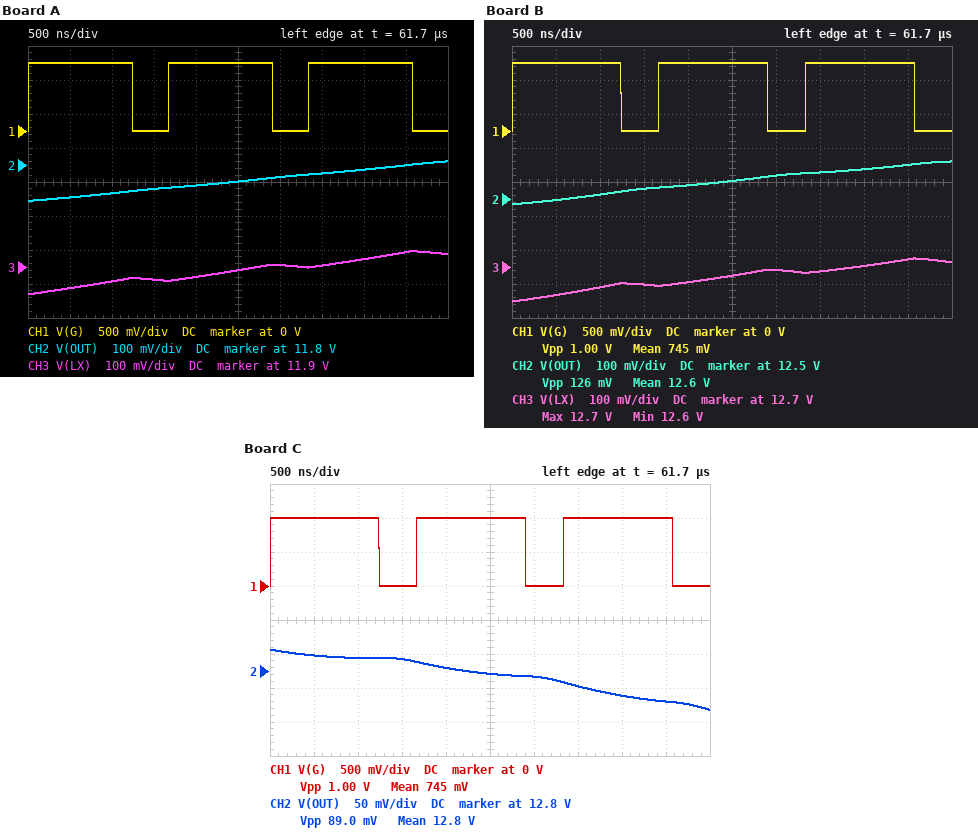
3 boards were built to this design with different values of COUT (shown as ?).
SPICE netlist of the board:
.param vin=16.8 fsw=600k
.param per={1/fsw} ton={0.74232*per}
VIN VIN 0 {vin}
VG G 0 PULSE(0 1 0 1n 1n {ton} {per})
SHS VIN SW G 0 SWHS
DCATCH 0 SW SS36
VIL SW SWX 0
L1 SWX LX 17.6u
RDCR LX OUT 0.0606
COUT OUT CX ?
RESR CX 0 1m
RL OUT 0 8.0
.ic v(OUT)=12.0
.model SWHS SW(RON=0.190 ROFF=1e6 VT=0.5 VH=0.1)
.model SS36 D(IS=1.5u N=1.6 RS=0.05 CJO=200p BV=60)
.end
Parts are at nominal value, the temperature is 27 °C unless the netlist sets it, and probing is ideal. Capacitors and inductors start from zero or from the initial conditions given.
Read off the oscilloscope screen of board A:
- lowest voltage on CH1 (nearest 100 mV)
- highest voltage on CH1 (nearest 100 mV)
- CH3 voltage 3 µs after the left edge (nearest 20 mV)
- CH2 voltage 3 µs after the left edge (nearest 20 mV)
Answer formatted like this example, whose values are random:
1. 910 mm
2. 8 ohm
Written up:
1. 0 V
2. 1.0 V
3. 11.90 V
4. 11.76 V
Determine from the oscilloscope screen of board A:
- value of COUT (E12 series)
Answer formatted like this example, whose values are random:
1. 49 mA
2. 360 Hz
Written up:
1. 33 µF
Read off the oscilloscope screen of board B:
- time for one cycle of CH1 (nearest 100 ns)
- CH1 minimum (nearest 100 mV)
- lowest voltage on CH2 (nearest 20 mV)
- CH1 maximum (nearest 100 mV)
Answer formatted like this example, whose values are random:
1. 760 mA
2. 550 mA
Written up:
1. 1.7 µs
2. 0 V
3. 12.48 V
4. 1.0 V
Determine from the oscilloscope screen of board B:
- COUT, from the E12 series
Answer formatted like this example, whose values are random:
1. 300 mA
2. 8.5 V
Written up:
1. 15 µF
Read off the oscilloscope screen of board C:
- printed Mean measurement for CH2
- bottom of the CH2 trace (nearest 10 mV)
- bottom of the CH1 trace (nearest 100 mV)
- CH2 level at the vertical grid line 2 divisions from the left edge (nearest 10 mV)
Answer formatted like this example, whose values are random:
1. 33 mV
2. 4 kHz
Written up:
1. 12.8 V
2. 12.74 V
3. 0 V
4. 12.82 V
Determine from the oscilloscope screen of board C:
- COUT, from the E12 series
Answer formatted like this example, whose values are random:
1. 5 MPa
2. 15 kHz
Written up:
1. 10 µF
